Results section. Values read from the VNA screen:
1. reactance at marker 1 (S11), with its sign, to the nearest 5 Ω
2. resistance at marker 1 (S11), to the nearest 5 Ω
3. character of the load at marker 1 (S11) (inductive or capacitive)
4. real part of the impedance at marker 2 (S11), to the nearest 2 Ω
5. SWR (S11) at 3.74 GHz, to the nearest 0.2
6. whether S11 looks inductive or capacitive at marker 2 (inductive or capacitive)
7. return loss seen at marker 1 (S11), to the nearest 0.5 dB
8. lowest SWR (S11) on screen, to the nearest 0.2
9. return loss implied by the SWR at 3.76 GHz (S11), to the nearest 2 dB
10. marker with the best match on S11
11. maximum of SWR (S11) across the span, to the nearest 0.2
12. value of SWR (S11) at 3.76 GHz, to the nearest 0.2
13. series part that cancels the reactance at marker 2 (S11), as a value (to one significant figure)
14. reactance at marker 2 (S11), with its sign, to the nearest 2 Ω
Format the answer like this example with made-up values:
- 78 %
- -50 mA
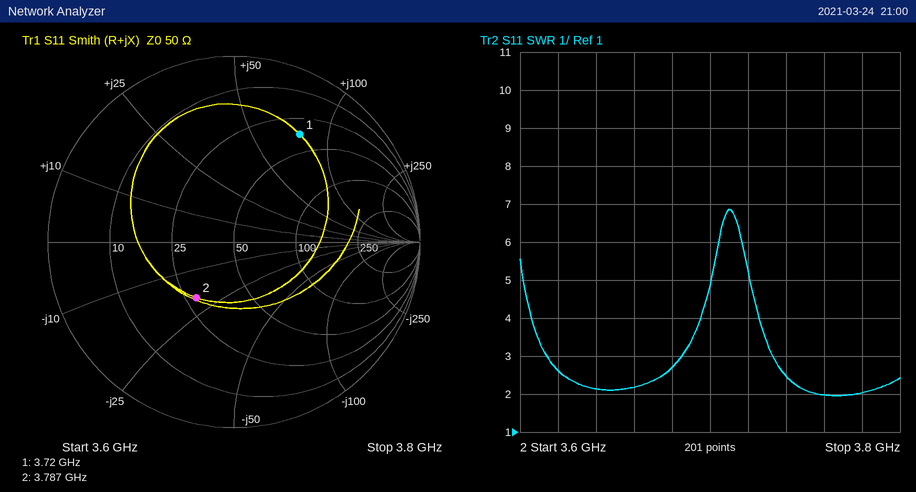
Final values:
- +75 Ω
- 35 Ω
- inductive
- 28 Ω
- 2.4
- capacitive
- 3.5 dB
- 2.0
- 10 dB
- marker 2
- 6.8
- 2.0
- 800 pH
- -20 Ω
